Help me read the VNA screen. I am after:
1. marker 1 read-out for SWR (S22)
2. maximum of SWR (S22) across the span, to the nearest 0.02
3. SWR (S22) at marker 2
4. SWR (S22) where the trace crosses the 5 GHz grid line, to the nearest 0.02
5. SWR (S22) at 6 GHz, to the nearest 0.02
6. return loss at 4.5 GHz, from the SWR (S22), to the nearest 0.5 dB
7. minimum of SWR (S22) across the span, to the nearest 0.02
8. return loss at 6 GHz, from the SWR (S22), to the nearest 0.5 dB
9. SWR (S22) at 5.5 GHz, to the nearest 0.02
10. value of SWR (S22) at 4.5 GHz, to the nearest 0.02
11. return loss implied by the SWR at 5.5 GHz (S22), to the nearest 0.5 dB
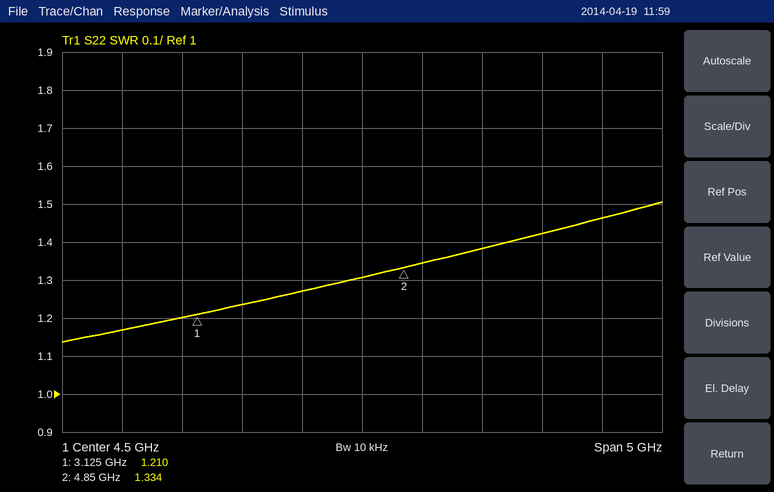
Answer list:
1.210
1.50
1.334
1.34
1.42
17.5 dB
1.14
15.0 dB
1.38
1.30
16.0 dB
